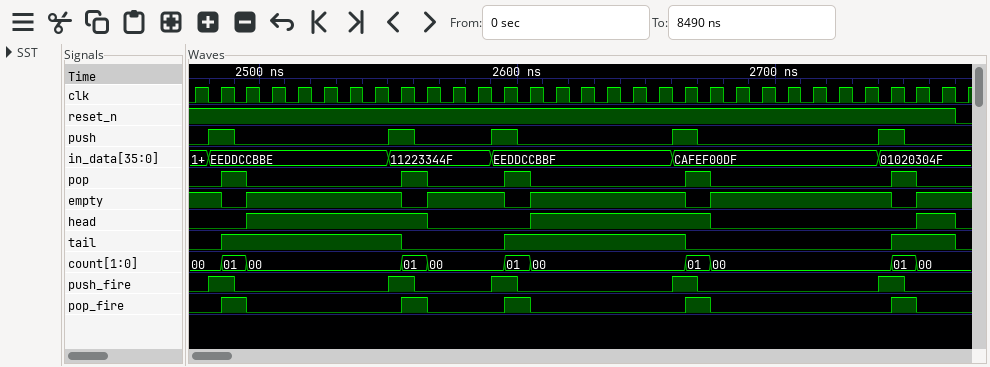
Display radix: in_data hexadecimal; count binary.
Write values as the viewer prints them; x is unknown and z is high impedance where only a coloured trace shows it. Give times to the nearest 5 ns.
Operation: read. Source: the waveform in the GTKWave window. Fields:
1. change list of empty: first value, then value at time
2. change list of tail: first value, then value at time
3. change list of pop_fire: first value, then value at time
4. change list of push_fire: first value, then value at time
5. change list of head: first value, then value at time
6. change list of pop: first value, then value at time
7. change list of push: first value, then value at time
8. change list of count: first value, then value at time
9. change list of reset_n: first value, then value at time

1, 0 at 2485 ns, 1 at 2495 ns, 0 at 2555 ns, 1 at 2565 ns, 0 at 2595 ns, 1 at 2605 ns, 0 at 2665 ns, 1 at 2675 ns, 0 at 2745 ns, 1 at 2755 ns
0, 1 at 2485 ns, 0 at 2555 ns, 1 at 2595 ns, 0 at 2665 ns, 1 at 2745 ns, 0 at 2770 ns
0, 1 at 2485 ns, 0 at 2495 ns, 1 at 2555 ns, 0 at 2565 ns, 1 at 2595 ns, 0 at 2605 ns, 1 at 2665 ns, 0 at 2675 ns, 1 at 2745 ns, 0 at 2755 ns
0, 1 at 2480 ns, 0 at 2490 ns, 1 at 2550 ns, 0 at 2560 ns, 1 at 2590 ns, 0 at 2600 ns, 1 at 2660 ns, 0 at 2670 ns, 1 at 2740 ns, 0 at 2750 ns
0, 1 at 2495 ns, 0 at 2565 ns, 1 at 2605 ns, 0 at 2675 ns, 1 at 2755 ns, 0 at 2770 ns
0, 1 at 2485 ns, 0 at 2495 ns, 1 at 2555 ns, 0 at 2565 ns, 1 at 2595 ns, 0 at 2605 ns, 1 at 2665 ns, 0 at 2675 ns, 1 at 2745 ns, 0 at 2755 ns
0, 1 at 2480 ns, 0 at 2490 ns, 1 at 2550 ns, 0 at 2560 ns, 1 at 2590 ns, 0 at 2600 ns, 1 at 2660 ns, 0 at 2670 ns, 1 at 2740 ns, 0 at 2750 ns
00, 01 at 2485 ns, 00 at 2495 ns, 01 at 2555 ns, 00 at 2565 ns, 01 at 2595 ns, 00 at 2605 ns, 01 at 2665 ns, 00 at 2675 ns, 01 at 2745 ns, 00 at 2755 ns
1, 0 at 2770 ns
